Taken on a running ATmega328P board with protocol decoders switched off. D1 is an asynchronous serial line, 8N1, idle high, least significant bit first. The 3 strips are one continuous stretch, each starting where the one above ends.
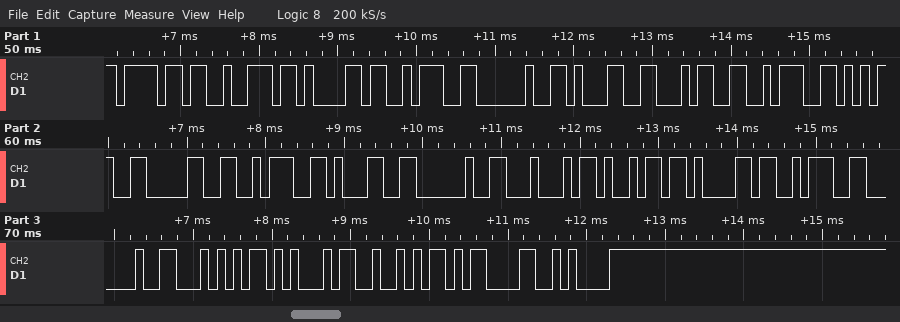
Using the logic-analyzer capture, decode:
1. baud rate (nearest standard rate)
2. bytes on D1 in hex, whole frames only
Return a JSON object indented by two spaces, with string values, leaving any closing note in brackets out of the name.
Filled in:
{
  "baud rate": "9600 baud",
  "bytes on D1 in hex, whole frames only": "6F 72 61 3A 20 31 34 3A 35 30 3A 31 20 44 69 61 3A 20 54 45 52 0D 0A"
}
